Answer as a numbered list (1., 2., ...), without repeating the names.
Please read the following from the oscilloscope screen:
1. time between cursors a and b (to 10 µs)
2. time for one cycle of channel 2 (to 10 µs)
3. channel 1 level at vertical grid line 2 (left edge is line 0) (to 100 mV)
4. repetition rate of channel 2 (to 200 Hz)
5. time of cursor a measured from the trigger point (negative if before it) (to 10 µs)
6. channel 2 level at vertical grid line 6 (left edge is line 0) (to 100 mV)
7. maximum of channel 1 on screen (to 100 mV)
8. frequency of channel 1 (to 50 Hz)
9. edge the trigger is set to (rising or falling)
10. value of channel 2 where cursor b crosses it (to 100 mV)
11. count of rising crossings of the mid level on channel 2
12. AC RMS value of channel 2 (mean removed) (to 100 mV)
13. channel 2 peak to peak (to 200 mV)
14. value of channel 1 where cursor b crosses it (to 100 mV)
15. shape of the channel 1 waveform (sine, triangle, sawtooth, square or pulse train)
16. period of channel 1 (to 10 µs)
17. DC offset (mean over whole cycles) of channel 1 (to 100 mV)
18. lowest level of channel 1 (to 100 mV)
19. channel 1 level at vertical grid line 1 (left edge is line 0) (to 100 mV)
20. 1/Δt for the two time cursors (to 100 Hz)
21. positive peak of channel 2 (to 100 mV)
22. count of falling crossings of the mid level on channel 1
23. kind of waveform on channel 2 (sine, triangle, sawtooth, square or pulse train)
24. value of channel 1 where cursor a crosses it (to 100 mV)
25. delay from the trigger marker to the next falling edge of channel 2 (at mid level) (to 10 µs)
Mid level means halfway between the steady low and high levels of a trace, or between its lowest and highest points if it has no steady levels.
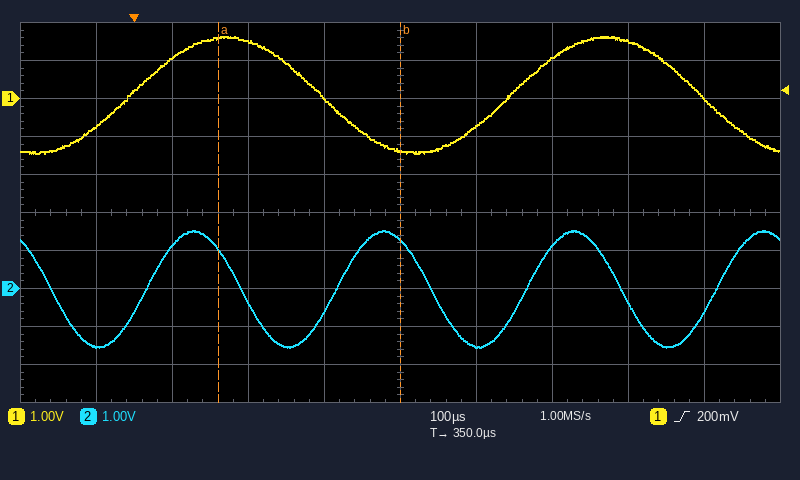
1. 240 µs
2. 250 µs
3. 1.1 V
4. 4.0 kHz
5. +110 µs
6. -1.5 V
7. 1.6 V
8. 2.00 kHz
9. rising
10. 1.3 V
11. 4
12. 1.1 V
13. 3.0 V
14. -1.4 V
15. sine
16. 500 µs
17. 100 mV
18. -1.4 V
19. -700 mV
20. 4.2 kHz
21. 1.5 V
22. 2
23. sine
24. 1.6 V
25. 140 µs
